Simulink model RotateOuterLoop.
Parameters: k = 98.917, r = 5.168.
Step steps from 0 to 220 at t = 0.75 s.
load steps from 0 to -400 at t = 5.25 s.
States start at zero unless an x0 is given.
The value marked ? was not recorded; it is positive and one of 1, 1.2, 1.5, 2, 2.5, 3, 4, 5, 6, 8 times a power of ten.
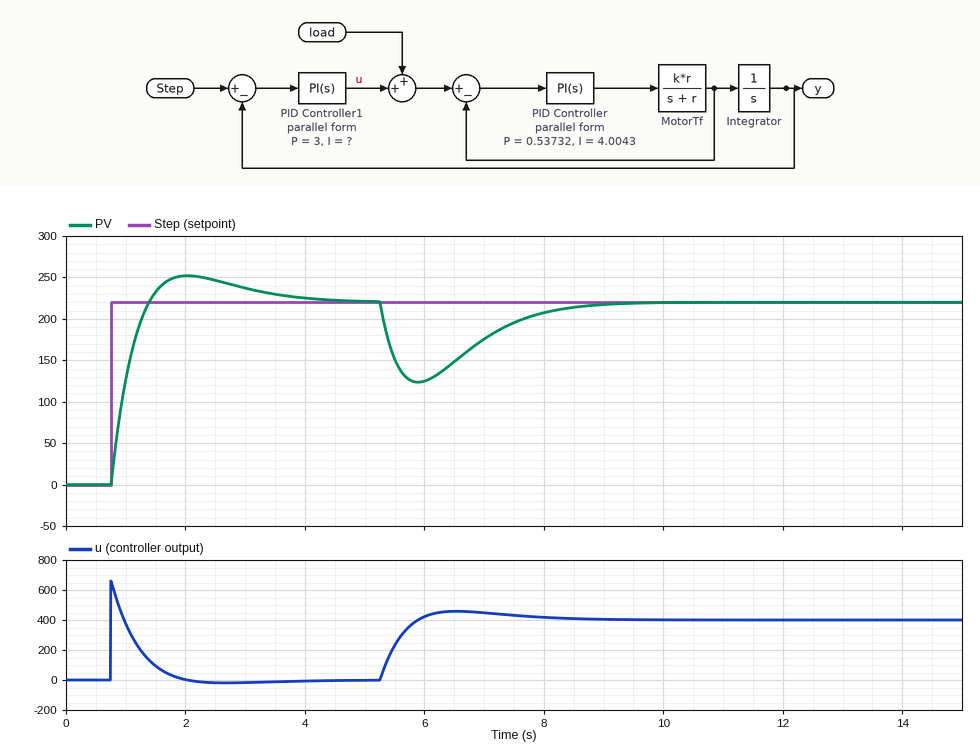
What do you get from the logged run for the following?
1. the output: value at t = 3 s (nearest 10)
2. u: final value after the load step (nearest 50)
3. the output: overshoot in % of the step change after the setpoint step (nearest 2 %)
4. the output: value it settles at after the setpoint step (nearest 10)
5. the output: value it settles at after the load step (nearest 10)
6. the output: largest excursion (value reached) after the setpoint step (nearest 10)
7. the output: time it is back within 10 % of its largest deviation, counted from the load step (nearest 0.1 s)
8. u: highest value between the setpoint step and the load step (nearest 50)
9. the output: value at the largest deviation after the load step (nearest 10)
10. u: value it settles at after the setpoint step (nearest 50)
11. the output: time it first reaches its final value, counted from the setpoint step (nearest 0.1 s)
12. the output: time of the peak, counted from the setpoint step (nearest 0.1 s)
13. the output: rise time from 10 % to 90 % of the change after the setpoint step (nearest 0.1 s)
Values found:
240
400
14 %
220
220
250
2.9 s
650
120
0
0.6 s
1.3 s
0.5 s
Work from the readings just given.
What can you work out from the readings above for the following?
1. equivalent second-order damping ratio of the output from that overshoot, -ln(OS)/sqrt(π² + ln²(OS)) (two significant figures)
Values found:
0.53
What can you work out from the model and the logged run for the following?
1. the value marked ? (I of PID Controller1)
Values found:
2.5
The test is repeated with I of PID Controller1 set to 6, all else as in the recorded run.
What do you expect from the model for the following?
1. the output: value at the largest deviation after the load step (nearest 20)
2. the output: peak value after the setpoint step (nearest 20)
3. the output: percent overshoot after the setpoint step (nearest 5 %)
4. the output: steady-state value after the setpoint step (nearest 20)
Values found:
140
280
25 %
220
